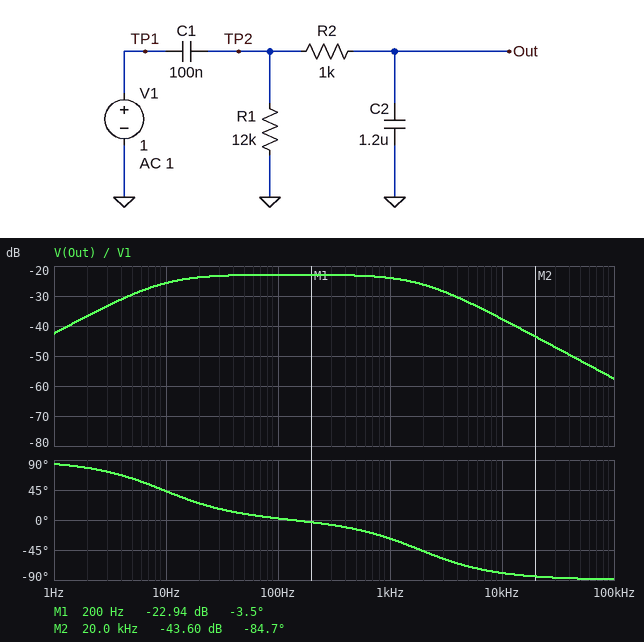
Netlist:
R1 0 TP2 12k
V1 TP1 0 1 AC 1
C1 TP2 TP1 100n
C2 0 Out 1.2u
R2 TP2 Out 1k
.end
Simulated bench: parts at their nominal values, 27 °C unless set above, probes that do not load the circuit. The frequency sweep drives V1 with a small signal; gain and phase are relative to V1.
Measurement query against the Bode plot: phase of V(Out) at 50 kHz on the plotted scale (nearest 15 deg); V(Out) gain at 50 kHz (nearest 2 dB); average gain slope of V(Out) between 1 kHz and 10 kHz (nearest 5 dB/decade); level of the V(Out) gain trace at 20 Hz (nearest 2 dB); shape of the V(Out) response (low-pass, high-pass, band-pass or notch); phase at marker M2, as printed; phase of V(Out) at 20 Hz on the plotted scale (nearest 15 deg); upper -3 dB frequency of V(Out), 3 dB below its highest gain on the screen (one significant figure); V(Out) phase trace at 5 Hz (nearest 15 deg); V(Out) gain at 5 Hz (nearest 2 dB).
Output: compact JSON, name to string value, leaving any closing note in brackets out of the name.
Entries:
{"phase of V(Out) at 50 kHz on the plotted scale": "-90 deg", "V(Out) gain at 50 kHz": "-52 dB", "average gain slope of V(Out) between 1 kHz and 10 kHz": "-15 dB/decade", "level of the V(Out) gain trace at 20 Hz": "-24 dB", "shape of the V(Out) response": "band-pass", "phase at marker M2, as printed": "-84.7 deg", "phase of V(Out) at 20 Hz on the plotted scale": "30 deg", "upper -3 dB frequency of V(Out), 3 dB below its highest gain on the screen": "2 kHz", "V(Out) phase trace at 5 Hz": "60 deg", "V(Out) gain at 5 Hz": "-30 dB"}
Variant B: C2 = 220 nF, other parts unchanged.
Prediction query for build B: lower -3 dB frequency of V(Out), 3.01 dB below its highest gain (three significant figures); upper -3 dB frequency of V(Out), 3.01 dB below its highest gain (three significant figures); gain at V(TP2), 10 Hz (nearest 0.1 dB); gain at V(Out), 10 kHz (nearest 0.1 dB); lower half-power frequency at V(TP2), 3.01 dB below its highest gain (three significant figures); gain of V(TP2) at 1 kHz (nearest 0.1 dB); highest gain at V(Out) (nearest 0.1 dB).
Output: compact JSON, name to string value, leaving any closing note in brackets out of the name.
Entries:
{"lower -3 dB frequency of V(Out), 3.01 dB below its highest gain": "38.6 Hz", "upper -3 dB frequency of V(Out), 3.01 dB below its highest gain": "2.49 kHz", "gain at V(TP2), 10 Hz": "-22.7 dB", "gain at V(Out), 10 kHz": "-23.1 dB", "lower half-power frequency at V(TP2), 3.01 dB below its highest gain": "2.18 kHz", "gain of V(TP2) at 1 kHz": "-6.5 dB", "highest gain at V(Out)": "-10.6 dB"}
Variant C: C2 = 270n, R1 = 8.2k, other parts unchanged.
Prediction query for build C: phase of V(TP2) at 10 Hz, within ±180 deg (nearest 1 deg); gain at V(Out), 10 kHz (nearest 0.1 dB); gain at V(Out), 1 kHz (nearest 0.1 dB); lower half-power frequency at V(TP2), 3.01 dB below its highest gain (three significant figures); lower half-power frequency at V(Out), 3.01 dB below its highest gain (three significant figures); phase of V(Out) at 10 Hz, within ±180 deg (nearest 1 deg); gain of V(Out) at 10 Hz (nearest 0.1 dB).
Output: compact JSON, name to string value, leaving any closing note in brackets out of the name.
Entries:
{"phase of V(TP2) at 10 Hz, within ±180 deg": "79 deg", "gain at V(Out), 10 kHz": "-24.8 dB", "gain at V(Out), 1 kHz": "-12.7 dB", "lower half-power frequency at V(TP2), 3.01 dB below its highest gain": "2.17 kHz", "lower half-power frequency at V(Out), 3.01 dB below its highest gain": "47.2 Hz", "phase of V(Out) at 10 Hz, within ±180 deg": "78 deg", "gain of V(Out) at 10 Hz": "-25.9 dB"}
